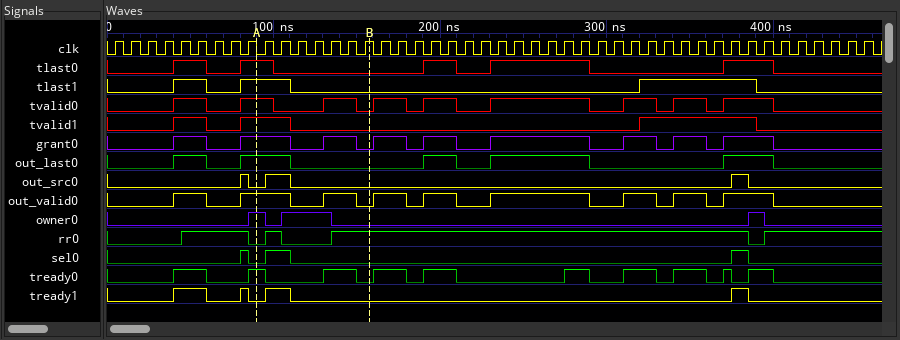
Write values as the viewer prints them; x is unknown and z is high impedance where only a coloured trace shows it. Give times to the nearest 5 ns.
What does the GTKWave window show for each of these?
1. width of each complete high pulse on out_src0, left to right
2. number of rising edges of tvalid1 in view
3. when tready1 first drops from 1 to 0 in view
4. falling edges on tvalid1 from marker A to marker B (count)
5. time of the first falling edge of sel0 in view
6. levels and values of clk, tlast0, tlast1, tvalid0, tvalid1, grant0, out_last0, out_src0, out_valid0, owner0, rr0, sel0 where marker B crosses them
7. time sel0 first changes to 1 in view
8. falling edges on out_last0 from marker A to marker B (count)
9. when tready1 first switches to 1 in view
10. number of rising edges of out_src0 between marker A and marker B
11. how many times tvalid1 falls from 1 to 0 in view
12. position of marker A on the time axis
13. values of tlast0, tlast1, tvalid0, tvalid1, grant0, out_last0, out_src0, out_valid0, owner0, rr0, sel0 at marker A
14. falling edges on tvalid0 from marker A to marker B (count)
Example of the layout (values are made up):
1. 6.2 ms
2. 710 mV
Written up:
1. 5 ns, 15 ns, 10 ns
2. 3
3. 60 ns
4. 1
5. 85 ns
6. clk=1, tlast0=0, tlast1=0, tvalid0=0, tvalid1=0, grant0=0, out_last0=0, out_src0=0, out_valid0=0, owner0=0, rr0=1, sel0=0
7. 80 ns
8. 1
9. 40 ns
10. 1
11. 3
12. 90 ns
13. tlast0=1, tlast1=1, tvalid0=1, tvalid1=1, grant0=1, out_last0=1, out_src0=0, out_valid0=1, owner0=1, rr0=0, sel0=0
14. 2
